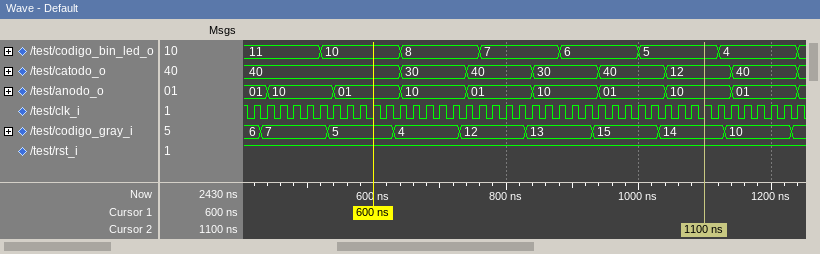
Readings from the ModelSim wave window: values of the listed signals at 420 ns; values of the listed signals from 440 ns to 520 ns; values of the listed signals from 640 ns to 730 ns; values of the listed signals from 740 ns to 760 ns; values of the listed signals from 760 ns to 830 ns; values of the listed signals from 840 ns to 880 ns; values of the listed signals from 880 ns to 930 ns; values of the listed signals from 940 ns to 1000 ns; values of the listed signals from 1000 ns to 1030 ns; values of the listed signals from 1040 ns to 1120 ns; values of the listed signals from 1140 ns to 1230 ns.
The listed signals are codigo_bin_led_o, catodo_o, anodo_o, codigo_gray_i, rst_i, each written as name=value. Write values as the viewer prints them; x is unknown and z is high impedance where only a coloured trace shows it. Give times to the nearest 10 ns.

codigo_bin_led_o=11, catodo_o=40, anodo_o=01, codigo_gray_i=6, rst_i=1
codigo_bin_led_o=11, catodo_o=40, anodo_o=10, codigo_gray_i=7, rst_i=1
codigo_bin_led_o=8, catodo_o=30, anodo_o=10, codigo_gray_i=4, rst_i=1
codigo_bin_led_o=8, catodo_o=40, anodo_o=01, codigo_gray_i=12, rst_i=1
codigo_bin_led_o=7, catodo_o=40, anodo_o=01, codigo_gray_i=12, rst_i=1
codigo_bin_led_o=7, catodo_o=30, anodo_o=10, codigo_gray_i=13, rst_i=1
codigo_bin_led_o=6, catodo_o=30, anodo_o=10, codigo_gray_i=13, rst_i=1
codigo_bin_led_o=6, catodo_o=40, anodo_o=01, codigo_gray_i=15, rst_i=1
codigo_bin_led_o=5, catodo_o=40, anodo_o=01, codigo_gray_i=15, rst_i=1
codigo_bin_led_o=5, catodo_o=12, anodo_o=10, codigo_gray_i=14, rst_i=1
codigo_bin_led_o=4, catodo_o=40, anodo_o=01, codigo_gray_i=10, rst_i=1
